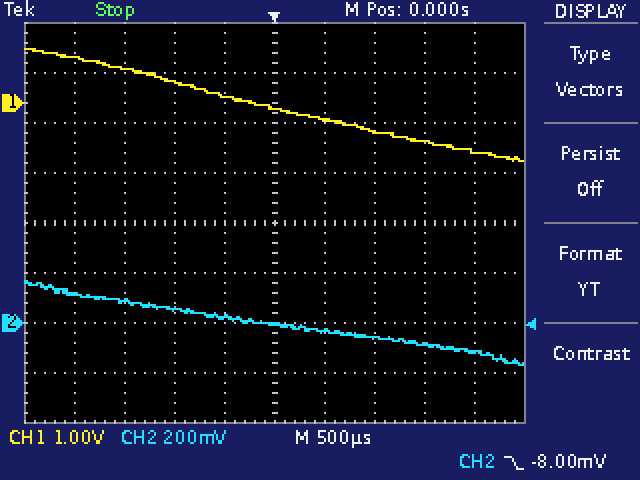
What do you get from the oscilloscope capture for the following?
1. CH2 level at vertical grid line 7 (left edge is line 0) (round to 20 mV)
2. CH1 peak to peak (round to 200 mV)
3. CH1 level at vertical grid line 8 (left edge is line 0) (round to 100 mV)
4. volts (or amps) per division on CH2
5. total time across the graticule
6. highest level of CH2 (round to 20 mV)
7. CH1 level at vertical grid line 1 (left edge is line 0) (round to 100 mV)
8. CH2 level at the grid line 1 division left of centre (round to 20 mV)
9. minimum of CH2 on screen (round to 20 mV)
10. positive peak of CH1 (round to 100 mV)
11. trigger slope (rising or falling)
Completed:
-60 mV
2.2 V
-800 mV
200 mV
5 ms
160 mV
900 mV
20 mV
-160 mV
1.1 V
falling
